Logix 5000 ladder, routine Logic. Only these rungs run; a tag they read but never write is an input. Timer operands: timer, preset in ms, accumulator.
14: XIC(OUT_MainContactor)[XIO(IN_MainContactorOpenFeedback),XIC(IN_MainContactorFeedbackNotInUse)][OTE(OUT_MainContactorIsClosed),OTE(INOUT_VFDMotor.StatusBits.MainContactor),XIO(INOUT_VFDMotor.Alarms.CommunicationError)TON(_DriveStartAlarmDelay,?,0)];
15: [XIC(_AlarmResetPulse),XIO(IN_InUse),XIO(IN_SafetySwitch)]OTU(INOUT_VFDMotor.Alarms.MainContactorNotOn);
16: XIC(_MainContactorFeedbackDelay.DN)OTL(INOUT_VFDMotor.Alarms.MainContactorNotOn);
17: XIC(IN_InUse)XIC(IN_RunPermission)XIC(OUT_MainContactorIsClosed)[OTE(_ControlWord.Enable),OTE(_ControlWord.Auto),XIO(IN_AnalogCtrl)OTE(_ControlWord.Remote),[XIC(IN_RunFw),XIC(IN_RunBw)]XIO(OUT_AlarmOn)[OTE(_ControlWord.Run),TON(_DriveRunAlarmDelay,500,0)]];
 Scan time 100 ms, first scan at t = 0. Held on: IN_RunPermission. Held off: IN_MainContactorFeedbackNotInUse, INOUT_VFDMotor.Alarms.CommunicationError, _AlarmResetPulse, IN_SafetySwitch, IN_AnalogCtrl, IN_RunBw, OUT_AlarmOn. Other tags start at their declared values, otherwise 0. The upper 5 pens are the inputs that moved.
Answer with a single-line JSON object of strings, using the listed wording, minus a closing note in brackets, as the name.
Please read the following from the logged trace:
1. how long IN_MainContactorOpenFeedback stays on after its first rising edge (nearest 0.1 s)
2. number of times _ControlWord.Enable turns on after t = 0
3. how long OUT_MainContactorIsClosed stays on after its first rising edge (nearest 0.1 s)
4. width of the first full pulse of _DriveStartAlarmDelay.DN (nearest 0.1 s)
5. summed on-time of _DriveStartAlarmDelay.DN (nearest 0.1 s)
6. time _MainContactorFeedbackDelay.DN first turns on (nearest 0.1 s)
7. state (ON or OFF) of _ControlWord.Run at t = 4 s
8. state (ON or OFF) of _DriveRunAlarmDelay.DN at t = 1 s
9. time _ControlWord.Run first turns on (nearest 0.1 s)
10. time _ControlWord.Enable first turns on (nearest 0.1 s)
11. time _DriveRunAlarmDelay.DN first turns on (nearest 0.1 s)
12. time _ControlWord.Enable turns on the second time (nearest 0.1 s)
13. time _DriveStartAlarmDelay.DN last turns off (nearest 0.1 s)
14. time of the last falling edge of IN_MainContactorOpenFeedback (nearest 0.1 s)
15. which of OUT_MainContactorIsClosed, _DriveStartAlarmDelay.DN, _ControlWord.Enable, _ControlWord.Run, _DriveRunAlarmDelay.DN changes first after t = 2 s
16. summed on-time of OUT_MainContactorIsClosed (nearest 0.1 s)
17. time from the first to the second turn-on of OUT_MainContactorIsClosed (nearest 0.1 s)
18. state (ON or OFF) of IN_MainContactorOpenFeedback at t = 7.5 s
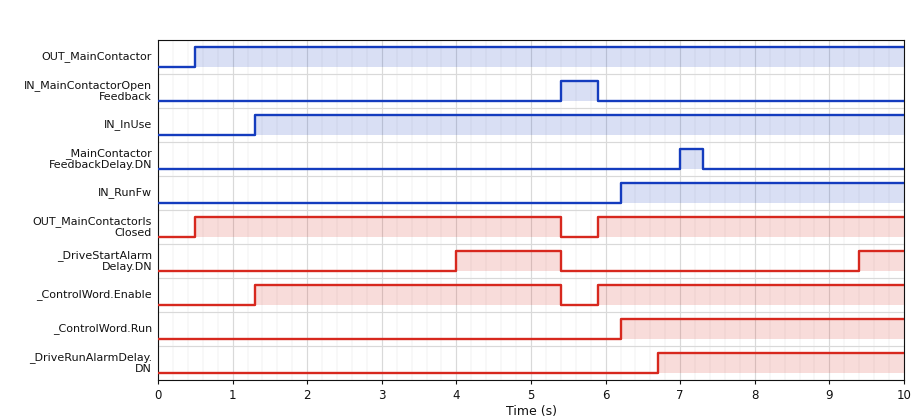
{"how long IN_MainContactorOpenFeedback stays on after its first rising edge": "0.5 s", "number of times _ControlWord.Enable turns on after t = 0": "2", "how long OUT_MainContactorIsClosed stays on after its first rising edge": "4.9 s", "width of the first full pulse of _DriveStartAlarmDelay.DN": "1.4 s", "summed on-time of _DriveStartAlarmDelay.DN": "2.0 s", "time _MainContactorFeedbackDelay.DN first turns on": "7.0 s", "state (ON or OFF) of _ControlWord.Run at t = 4 s": "OFF", "state (ON or OFF) of _DriveRunAlarmDelay.DN at t = 1 s": "OFF", "time _ControlWord.Run first turns on": "6.2 s", "time _ControlWord.Enable first turns on": "1.3 s", "time _DriveRunAlarmDelay.DN first turns on": "6.7 s", "time _ControlWord.Enable turns on the second time": "5.9 s", "time _DriveStartAlarmDelay.DN last turns off": "5.4 s", "time of the last falling edge of IN_MainContactorOpenFeedback": "5.9 s", "which of OUT_MainContactorIsClosed, _DriveStartAlarmDelay.DN, _ControlWord.Enable, _ControlWord.Run, _DriveRunAlarmDelay.DN changes first after t = 2 s": "_DriveStartAlarmDelay.DN", "summed on-time of OUT_MainContactorIsClosed": "9.0 s", "time from the first to the second turn-on of OUT_MainContactorIsClosed": "5.4 s", "state (ON or OFF) of IN_MainContactorOpenFeedback at t = 7.5 s": "OFF"}
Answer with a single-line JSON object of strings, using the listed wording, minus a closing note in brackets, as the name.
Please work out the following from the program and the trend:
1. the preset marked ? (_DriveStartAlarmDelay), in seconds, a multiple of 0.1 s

{"the preset marked ? (_DriveStartAlarmDelay), in seconds, a multiple of 0.1 s": "3.5 s"}
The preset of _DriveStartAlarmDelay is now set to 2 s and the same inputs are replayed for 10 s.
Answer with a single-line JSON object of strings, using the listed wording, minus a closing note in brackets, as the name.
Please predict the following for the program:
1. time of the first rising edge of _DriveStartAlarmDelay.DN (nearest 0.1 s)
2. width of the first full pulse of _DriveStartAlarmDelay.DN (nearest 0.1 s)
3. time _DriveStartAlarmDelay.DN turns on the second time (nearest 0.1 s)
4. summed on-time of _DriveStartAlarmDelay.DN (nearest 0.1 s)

{"time of the first rising edge of _DriveStartAlarmDelay.DN": "2.5 s", "width of the first full pulse of _DriveStartAlarmDelay.DN": "2.9 s", "time _DriveStartAlarmDelay.DN turns on the second time": "7.9 s", "summed on-time of _DriveStartAlarmDelay.DN": "5.0 s"}
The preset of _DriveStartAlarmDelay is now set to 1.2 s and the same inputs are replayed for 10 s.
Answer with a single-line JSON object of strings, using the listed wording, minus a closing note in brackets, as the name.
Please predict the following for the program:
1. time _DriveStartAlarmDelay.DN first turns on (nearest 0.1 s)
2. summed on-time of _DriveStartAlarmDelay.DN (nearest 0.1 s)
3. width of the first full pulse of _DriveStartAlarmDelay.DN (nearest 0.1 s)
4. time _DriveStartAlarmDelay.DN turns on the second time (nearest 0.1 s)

{"time _DriveStartAlarmDelay.DN first turns on": "1.7 s", "summed on-time of _DriveStartAlarmDelay.DN": "6.6 s", "width of the first full pulse of _DriveStartAlarmDelay.DN": "3.7 s", "time _DriveStartAlarmDelay.DN turns on the second time": "7.1 s"}
